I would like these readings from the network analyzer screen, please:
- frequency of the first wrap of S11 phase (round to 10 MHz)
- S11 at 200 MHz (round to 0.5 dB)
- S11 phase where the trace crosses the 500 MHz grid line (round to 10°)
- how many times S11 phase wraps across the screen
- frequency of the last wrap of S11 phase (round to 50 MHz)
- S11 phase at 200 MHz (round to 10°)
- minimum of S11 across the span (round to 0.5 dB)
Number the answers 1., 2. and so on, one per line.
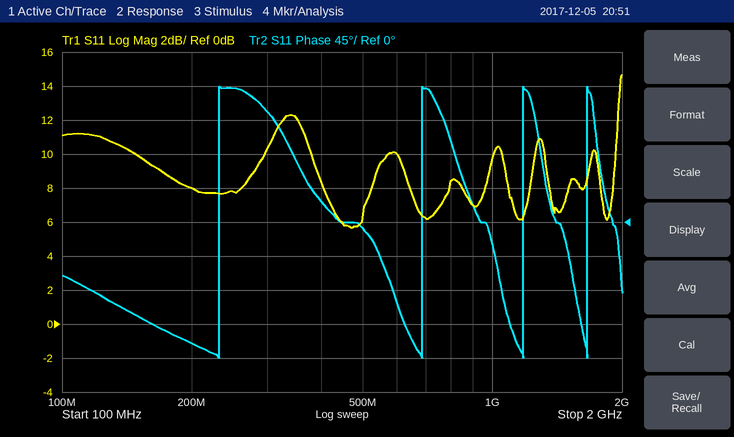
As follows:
1. 230 MHz
2. 8.0 dB
3. -10°
4. 4
5. 1.65 GHz
6. -160°
7. 5.5 dB
